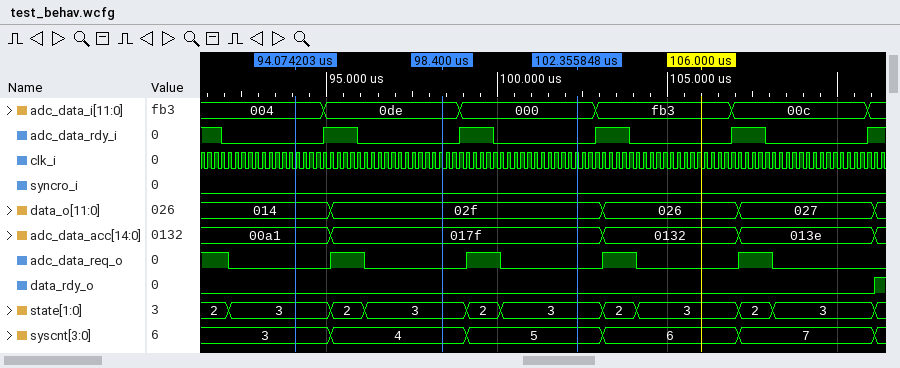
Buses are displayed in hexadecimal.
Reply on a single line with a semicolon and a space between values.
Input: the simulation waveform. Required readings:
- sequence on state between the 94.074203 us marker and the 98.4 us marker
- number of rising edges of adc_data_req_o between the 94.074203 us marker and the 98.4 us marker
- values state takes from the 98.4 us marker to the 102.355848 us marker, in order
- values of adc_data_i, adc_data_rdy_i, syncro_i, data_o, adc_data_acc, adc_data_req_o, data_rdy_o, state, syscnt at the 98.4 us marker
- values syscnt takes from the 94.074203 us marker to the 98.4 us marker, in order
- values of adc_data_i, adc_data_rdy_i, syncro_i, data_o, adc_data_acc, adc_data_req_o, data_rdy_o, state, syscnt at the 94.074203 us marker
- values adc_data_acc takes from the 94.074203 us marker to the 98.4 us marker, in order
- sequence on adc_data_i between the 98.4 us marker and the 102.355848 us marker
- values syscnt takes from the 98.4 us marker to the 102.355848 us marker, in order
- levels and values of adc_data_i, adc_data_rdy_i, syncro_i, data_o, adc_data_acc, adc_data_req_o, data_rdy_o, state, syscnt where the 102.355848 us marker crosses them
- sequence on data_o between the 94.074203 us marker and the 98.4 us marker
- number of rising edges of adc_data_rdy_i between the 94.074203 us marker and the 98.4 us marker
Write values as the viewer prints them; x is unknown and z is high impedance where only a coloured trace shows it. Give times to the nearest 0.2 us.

3, 2, 3; 1; 3, 2, 3; adc_data_i=0de, adc_data_rdy_i=0, syncro_i=0, data_o=02f, adc_data_acc=017f, adc_data_req_o=0, data_rdy_o=0, state=3, syscnt=4; 3, 4; adc_data_i=004, adc_data_rdy_i=0, syncro_i=0, data_o=014, adc_data_acc=00a1, adc_data_req_o=0, data_rdy_o=0, state=3, syscnt=3; 00a1, 017f; 0de, 000; 4, 5; adc_data_i=000, adc_data_rdy_i=0, syncro_i=0, data_o=02f, adc_data_acc=017f, adc_data_req_o=0, data_rdy_o=0, state=3, syscnt=5; 014, 02f; 1
